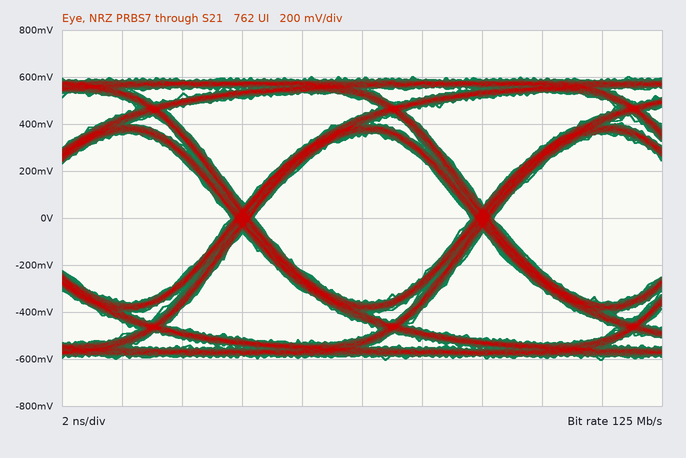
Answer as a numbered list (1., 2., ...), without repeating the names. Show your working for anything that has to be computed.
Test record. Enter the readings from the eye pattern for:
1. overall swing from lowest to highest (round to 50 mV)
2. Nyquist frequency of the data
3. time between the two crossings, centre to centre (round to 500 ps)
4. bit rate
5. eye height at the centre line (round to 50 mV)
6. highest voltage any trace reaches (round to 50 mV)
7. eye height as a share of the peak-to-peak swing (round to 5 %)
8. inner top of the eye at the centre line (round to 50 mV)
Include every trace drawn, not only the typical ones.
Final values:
1. 1.20 V
2. 62.5 MHz
3. 8.0 ns
4. 125 Mb/s
5. 700 mV
6. 600 mV
7. 700 mV / 1.20 V ≈ 58.3 %, so 60 % to the nearest 5 %
8. 350 mV
